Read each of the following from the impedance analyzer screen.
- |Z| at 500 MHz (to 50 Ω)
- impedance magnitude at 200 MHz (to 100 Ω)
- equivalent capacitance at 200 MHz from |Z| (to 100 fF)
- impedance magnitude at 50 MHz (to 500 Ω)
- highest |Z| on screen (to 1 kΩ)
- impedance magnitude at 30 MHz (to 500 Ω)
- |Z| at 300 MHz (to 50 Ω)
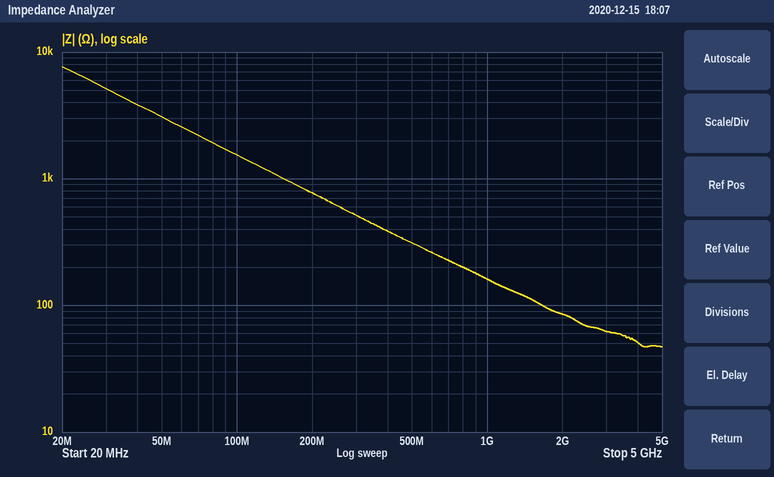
300 Ω
800 Ω
1.0 pF
3.0 kΩ
8 kΩ
5.0 kΩ
500 Ω
